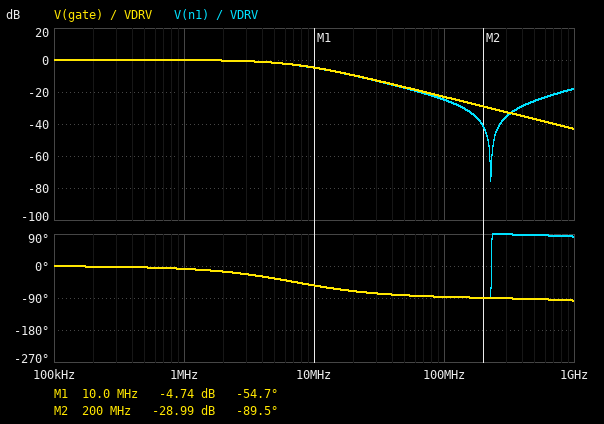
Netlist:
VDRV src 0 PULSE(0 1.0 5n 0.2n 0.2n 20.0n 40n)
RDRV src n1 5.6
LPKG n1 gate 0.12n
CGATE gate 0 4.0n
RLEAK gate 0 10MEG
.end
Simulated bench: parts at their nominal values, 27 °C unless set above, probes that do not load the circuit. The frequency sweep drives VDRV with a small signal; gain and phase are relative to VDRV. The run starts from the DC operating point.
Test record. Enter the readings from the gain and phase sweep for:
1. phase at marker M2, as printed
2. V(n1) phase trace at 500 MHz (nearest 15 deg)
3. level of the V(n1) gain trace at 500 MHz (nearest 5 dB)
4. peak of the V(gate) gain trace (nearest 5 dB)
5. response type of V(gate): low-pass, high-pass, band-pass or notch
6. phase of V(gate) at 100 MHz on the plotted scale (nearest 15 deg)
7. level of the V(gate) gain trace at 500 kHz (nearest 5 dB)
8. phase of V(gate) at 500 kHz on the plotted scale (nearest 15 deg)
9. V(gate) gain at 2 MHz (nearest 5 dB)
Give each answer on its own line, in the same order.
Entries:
-89.5 deg
90 deg
-25 dB
0 dB
low-pass
-90 deg
0 dB
0 deg
0 dB
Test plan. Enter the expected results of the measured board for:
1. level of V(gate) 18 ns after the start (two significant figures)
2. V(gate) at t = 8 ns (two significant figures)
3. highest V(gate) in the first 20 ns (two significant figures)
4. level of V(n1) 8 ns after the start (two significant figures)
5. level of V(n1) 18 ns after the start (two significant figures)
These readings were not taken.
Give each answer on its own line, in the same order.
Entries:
440 mV
120 mV
490 mV
120 mV
440 mV
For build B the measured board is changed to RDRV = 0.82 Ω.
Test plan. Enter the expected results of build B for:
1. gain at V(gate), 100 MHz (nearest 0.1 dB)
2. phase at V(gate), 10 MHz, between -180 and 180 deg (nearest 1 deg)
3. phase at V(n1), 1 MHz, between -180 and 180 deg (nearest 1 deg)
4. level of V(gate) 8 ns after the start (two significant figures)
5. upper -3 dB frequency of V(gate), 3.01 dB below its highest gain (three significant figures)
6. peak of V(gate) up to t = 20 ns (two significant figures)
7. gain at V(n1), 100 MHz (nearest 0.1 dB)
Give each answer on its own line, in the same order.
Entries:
-6.9 dB
-12 deg
-1 deg
580 mV
50.8 MHz
990 mV
-8.7 dB
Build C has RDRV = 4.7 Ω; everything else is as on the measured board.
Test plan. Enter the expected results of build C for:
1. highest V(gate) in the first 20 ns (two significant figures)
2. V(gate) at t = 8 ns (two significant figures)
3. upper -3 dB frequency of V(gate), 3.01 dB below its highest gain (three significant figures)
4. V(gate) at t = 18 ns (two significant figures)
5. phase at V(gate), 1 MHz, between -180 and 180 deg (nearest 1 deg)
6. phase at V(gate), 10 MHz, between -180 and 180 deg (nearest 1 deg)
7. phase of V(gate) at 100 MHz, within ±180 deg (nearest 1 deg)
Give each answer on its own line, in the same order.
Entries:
550 mV
140 mV
8.48 MHz
500 mV
-7 deg
-50 deg
-86 deg
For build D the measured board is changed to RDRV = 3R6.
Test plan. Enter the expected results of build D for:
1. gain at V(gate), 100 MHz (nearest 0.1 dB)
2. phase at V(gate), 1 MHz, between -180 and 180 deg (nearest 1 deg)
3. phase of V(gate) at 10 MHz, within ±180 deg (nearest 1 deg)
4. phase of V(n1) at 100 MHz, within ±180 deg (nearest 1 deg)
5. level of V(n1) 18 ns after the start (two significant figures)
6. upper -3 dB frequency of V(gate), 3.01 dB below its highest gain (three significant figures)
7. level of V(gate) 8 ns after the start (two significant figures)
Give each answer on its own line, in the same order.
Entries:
-19.2 dB
-5 deg
-42 deg
-85 deg
590 mV
11.1 MHz
180 mV
